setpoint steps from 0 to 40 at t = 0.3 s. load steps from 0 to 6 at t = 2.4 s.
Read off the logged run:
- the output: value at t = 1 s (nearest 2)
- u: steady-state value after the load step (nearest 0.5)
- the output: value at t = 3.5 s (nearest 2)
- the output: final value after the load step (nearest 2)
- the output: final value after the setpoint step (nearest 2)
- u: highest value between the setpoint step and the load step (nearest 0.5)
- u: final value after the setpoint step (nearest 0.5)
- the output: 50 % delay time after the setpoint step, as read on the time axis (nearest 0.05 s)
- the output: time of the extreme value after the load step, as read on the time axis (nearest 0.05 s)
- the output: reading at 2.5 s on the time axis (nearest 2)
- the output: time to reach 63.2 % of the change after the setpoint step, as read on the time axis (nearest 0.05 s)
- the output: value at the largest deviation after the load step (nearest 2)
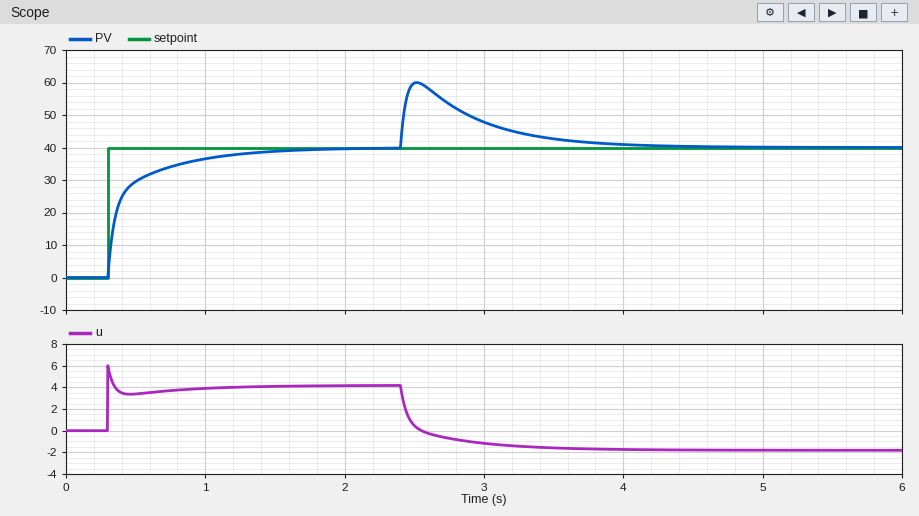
36
-2.0
42
40
40
6.0
4.0
0.35 s
2.50 s
60
0.40 s
60
